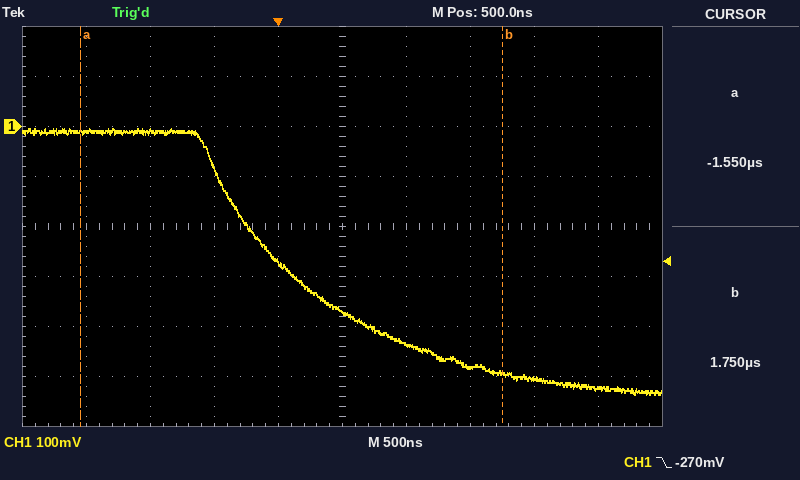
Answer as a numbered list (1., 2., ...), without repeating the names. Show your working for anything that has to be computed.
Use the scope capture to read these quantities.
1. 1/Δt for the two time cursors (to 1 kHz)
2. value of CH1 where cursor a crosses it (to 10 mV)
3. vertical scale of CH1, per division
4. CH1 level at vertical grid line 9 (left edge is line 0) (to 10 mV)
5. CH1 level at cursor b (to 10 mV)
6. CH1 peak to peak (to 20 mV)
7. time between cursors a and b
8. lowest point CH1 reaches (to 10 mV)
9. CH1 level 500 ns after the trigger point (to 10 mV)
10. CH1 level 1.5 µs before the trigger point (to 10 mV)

1. 1 / 3.30 µs ≈ 303 kHz
2. -10 mV
3. 100 mV
4. -520 mV
5. -490 mV
6. 540 mV
7. 1.75 µs − (-1.55 µs) = 3.30 µs
8. -540 mV
9. -370 mV
10. -10 mV
